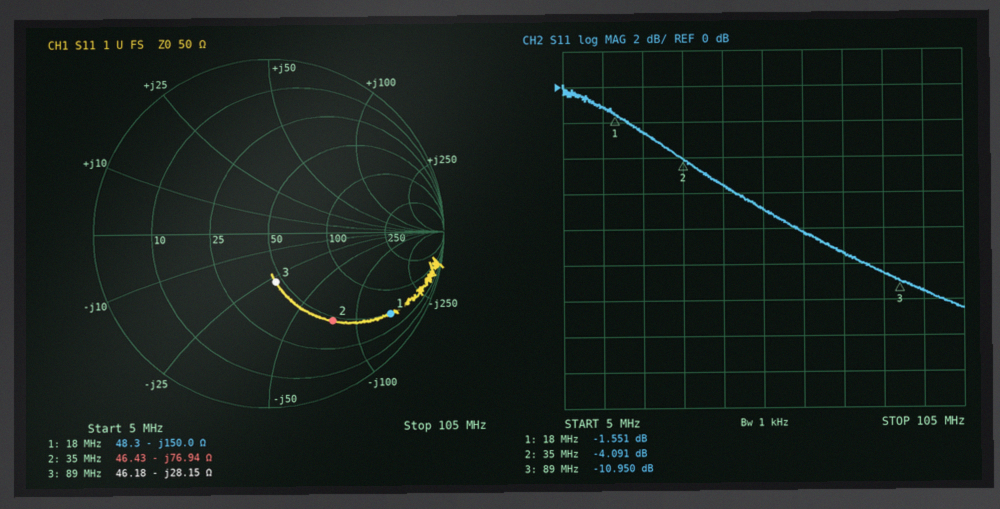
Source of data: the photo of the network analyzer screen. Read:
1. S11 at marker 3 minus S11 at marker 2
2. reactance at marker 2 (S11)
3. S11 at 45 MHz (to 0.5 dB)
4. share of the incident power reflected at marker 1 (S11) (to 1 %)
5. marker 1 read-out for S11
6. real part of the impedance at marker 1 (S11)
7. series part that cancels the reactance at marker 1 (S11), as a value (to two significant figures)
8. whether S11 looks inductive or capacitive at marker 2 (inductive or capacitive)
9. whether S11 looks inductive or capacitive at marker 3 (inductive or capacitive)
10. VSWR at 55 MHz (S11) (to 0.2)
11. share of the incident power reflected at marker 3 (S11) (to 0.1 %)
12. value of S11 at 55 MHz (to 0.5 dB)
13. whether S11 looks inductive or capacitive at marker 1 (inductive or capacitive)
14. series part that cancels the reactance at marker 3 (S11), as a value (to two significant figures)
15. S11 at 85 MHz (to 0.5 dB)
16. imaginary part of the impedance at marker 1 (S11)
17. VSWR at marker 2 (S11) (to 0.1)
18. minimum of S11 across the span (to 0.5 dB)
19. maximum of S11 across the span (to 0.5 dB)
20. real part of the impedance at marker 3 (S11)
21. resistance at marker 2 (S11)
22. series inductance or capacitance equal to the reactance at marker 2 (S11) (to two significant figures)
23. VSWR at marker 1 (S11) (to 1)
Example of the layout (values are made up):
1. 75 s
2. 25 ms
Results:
1. -6.859 dB
2. -76.94 Ω
3. -5.5 dB
4. 70 %
5. -1.551 dB
6. 48.3 Ω
7. 1.3 µH
8. capacitive
9. capacitive
10. 2.6
11. 8.0 %
12. -7.0 dB
13. capacitive
14. 50 nH
15. -10.5 dB
16. -150.0 Ω
17. 4.3
18. -12.5 dB
19. 0.0 dB
20. 46.18 Ω
21. 46.43 Ω
22. 59 pF
23. 11
